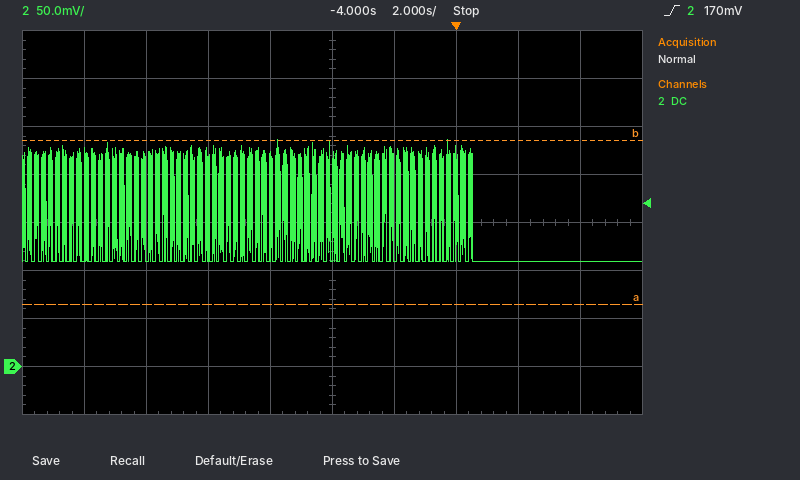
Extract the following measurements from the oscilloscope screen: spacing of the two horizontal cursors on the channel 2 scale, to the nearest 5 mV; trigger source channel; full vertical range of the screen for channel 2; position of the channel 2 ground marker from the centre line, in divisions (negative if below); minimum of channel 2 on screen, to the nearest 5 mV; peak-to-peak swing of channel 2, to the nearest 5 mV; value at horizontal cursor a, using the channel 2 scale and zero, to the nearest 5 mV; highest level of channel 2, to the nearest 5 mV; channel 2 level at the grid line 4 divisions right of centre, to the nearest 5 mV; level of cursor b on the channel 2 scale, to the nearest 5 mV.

170 mV
channel 2
400 mV
-3.0 div
110 mV
125 mV
65 mV
235 mV
110 mV
235 mV
